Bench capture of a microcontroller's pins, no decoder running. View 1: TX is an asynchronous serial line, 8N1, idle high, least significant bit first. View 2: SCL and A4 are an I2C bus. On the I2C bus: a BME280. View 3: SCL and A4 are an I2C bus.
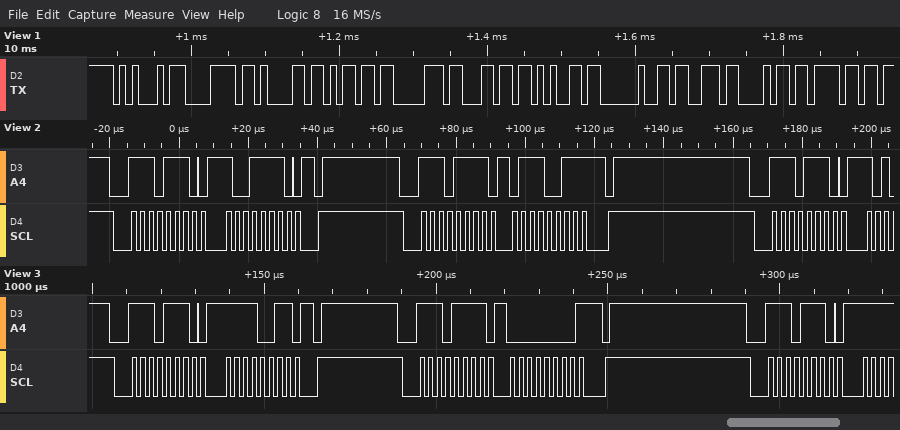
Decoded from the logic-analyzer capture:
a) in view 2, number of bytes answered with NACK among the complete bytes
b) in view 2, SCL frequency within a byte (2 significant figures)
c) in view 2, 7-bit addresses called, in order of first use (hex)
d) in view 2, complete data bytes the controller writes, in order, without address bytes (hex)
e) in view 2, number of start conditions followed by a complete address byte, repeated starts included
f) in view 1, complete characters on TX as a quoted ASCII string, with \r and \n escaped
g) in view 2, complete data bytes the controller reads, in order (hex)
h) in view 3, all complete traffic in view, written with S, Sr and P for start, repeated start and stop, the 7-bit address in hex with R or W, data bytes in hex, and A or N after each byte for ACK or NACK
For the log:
1
400 kHz
0x77
9E
3
"Example sho"
73
S 77W A F3 A P S 77R A 00 N P S 77W A
